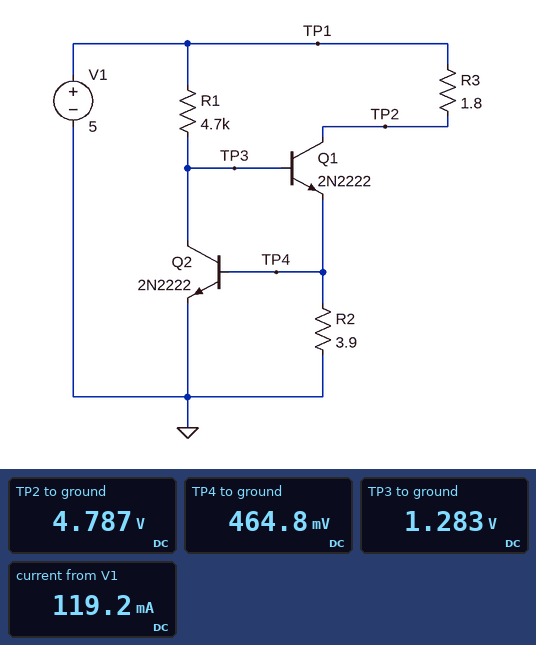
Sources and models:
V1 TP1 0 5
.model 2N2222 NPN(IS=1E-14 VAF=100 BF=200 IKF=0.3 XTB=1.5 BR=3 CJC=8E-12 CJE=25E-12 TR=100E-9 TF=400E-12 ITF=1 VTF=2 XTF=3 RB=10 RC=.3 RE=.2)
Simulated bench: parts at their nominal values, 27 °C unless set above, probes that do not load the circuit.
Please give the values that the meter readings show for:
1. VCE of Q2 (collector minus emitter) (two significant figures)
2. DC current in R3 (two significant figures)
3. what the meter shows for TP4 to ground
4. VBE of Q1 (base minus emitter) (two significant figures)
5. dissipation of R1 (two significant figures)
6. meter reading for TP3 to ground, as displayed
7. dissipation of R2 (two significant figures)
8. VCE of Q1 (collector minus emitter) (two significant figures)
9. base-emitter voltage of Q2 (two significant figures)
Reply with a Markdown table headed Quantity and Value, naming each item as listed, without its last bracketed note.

| Quantity | Value |
|---|---|
| VCE of Q2 (collector minus emitter) | 1.3 V |
| DC current in R3 | 120 mA |
| what the meter shows for TP4 to ground | 464.8 mV |
| VBE of Q1 (base minus emitter) | 820 mV |
| dissipation of R1 | 2.9 mW |
| meter reading for TP3 to ground, as displayed | 1.283 V |
| dissipation of R2 | 55 mW |
| VCE of Q1 (collector minus emitter) | 4.3 V |
| base-emitter voltage of Q2 | 460 mV |
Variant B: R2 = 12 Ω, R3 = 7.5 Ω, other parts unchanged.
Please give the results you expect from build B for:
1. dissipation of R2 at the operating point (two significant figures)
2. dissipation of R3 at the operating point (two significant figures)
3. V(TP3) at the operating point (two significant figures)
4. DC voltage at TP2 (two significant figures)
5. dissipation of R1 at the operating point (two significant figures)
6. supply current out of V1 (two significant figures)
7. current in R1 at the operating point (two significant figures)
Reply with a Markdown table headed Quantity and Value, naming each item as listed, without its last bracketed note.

| Quantity | Value |
|---|---|
| dissipation of R2 at the operating point | 34 mW |
| dissipation of R3 at the operating point | 21 mW |
| V(TP3) at the operating point | 1.4 V |
| DC voltage at TP2 | 4.6 V |
| dissipation of R1 at the operating point | 2.7 mW |
| supply current out of V1 | 53 mA |
| current in R1 at the operating point | 760 µA |
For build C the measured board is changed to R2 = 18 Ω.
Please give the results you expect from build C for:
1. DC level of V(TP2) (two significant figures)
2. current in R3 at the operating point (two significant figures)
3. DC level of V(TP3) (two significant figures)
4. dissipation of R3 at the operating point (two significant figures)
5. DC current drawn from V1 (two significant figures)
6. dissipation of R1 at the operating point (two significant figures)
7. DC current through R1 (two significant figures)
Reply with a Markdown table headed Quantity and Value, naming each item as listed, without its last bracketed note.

| Quantity | Value |
|---|---|
| DC level of V(TP2) | 4.9 V |
| current in R3 at the operating point | 35 mA |
| DC level of V(TP3) | 1.4 V |
| dissipation of R3 at the operating point | 2.3 mW |
| DC current drawn from V1 | 36 mA |
| dissipation of R1 at the operating point | 2.8 mW |
| DC current through R1 | 770 µA |
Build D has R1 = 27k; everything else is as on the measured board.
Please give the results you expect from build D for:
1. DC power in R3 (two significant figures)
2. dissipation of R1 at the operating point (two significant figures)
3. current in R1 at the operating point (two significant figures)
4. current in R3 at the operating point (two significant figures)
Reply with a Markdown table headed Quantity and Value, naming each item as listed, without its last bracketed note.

| Quantity | Value |
|---|---|
| DC power in R3 | 1.5 mW |
| dissipation of R1 at the operating point | 630 µW |
| current in R1 at the operating point | 150 µA |
| current in R3 at the operating point | 29 mA |
